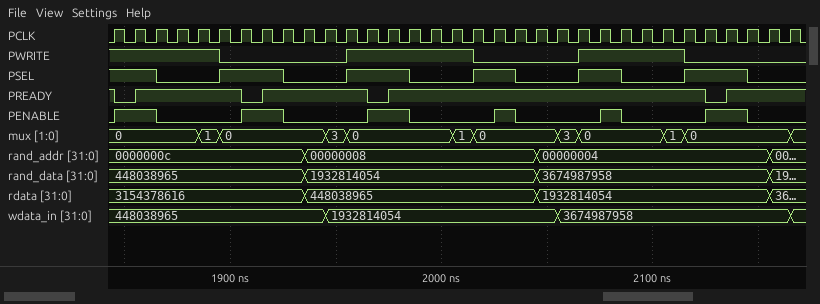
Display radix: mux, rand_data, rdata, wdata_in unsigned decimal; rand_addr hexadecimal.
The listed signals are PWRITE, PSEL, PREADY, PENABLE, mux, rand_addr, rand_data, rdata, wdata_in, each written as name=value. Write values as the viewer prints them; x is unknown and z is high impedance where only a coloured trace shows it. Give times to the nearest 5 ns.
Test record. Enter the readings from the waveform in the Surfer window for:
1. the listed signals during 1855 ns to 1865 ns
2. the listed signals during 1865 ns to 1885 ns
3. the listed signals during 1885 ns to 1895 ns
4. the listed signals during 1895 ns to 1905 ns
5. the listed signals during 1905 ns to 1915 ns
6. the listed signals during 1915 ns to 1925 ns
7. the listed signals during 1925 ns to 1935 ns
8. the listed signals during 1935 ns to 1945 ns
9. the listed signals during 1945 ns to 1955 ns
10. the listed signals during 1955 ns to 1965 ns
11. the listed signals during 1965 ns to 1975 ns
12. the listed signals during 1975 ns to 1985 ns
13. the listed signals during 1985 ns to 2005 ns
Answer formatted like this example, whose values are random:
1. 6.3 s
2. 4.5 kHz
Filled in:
1. PWRITE=1, PSEL=1, PREADY=1, PENABLE=1, mux=0, rand_addr=0000000c, rand_data=448038965, rdata=3154378616, wdata_in=448038965
2. PWRITE=1, PSEL=0, PREADY=1, PENABLE=0, mux=0, rand_addr=0000000c, rand_data=448038965, rdata=3154378616, wdata_in=448038965
3. PWRITE=1, PSEL=0, PREADY=1, PENABLE=0, mux=1, rand_addr=0000000c, rand_data=448038965, rdata=3154378616, wdata_in=448038965
4. PWRITE=0, PSEL=1, PREADY=1, PENABLE=0, mux=0, rand_addr=0000000c, rand_data=448038965, rdata=3154378616, wdata_in=448038965
5. PWRITE=0, PSEL=1, PREADY=0, PENABLE=1, mux=0, rand_addr=0000000c, rand_data=448038965, rdata=3154378616, wdata_in=448038965
6. PWRITE=0, PSEL=1, PREADY=1, PENABLE=1, mux=0, rand_addr=0000000c, rand_data=448038965, rdata=3154378616, wdata_in=448038965
7. PWRITE=0, PSEL=0, PREADY=1, PENABLE=0, mux=0, rand_addr=0000000c, rand_data=448038965, rdata=3154378616, wdata_in=448038965
8. PWRITE=0, PSEL=0, PREADY=1, PENABLE=0, mux=0, rand_addr=00000008, rand_data=1932814054, rdata=448038965, wdata_in=448038965
9. PWRITE=0, PSEL=0, PREADY=1, PENABLE=0, mux=3, rand_addr=00000008, rand_data=1932814054, rdata=448038965, wdata_in=1932814054
10. PWRITE=1, PSEL=1, PREADY=1, PENABLE=0, mux=0, rand_addr=00000008, rand_data=1932814054, rdata=448038965, wdata_in=1932814054
11. PWRITE=1, PSEL=1, PREADY=0, PENABLE=1, mux=0, rand_addr=00000008, rand_data=1932814054, rdata=448038965, wdata_in=1932814054
12. PWRITE=1, PSEL=1, PREADY=1, PENABLE=1, mux=0, rand_addr=00000008, rand_data=1932814054, rdata=448038965, wdata_in=1932814054
13. PWRITE=1, PSEL=0, PREADY=1, PENABLE=0, mux=0, rand_addr=00000008, rand_data=1932814054, rdata=448038965, wdata_in=1932814054
